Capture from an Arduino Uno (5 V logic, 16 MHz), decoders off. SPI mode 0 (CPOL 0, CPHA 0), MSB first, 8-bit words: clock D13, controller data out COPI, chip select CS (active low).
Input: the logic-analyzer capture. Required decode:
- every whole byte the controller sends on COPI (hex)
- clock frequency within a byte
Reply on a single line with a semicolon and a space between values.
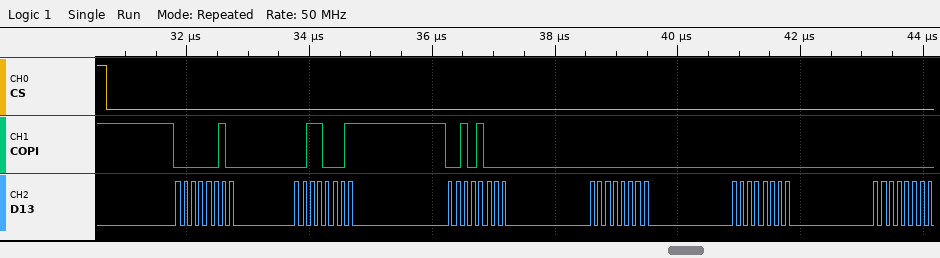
0x02 0x31 0x28 0x00 0x00 0x00; 8 MHz
